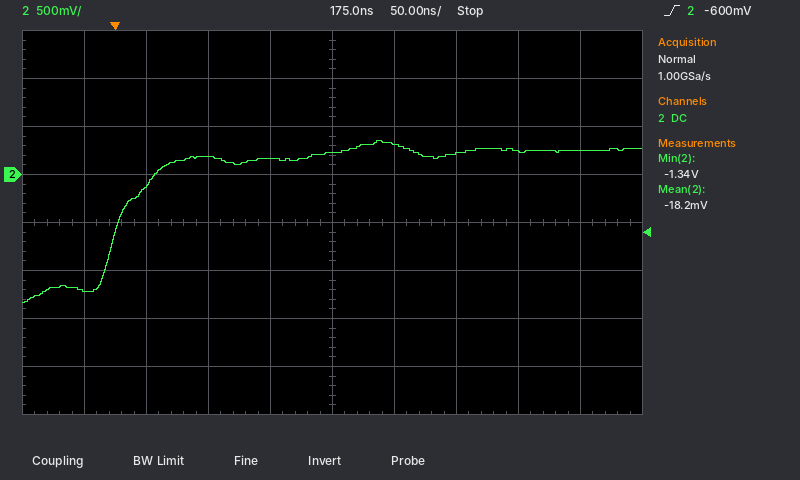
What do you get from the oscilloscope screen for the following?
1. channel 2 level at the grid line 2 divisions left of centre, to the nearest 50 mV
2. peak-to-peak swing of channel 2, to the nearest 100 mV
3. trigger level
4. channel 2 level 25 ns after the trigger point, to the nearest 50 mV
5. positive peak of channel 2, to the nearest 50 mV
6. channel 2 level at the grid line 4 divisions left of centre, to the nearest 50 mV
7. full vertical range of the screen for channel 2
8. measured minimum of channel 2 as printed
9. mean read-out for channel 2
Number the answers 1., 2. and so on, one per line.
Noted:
1. 200 mV
2. 1.70 V
3. -600 mV
4. -100 mV
5. 350 mV
6. -1.20 V
7. 4 V
8. -1.34 V
9. -18.2 mV
